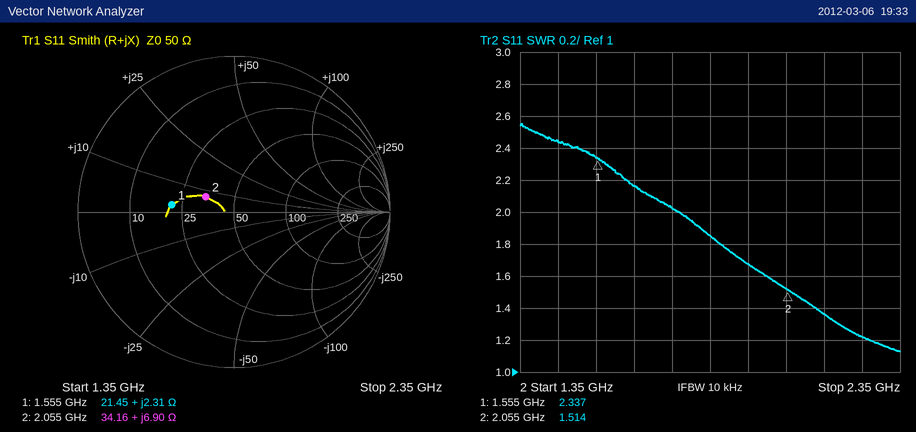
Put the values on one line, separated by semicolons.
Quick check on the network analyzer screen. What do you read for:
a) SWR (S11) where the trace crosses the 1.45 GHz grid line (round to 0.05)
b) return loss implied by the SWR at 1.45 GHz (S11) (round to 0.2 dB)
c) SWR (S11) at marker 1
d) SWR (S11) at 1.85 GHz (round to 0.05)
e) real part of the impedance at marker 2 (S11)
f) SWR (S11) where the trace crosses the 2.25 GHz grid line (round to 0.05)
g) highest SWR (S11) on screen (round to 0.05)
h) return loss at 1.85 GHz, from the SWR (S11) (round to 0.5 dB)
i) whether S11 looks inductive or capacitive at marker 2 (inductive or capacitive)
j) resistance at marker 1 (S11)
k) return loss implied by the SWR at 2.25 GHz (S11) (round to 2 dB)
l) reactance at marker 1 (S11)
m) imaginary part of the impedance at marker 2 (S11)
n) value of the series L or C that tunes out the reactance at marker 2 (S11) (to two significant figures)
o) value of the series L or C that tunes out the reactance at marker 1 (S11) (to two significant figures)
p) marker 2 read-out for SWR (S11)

2.45; 7.6 dB; 2.337; 1.85; 34.16 Ω; 1.20; 2.55; 10.5 dB; inductive; 21.45 Ω; 20 dB; +2.31 Ω; +6.90 Ω; 11 pF; 44 pF; 1.514
